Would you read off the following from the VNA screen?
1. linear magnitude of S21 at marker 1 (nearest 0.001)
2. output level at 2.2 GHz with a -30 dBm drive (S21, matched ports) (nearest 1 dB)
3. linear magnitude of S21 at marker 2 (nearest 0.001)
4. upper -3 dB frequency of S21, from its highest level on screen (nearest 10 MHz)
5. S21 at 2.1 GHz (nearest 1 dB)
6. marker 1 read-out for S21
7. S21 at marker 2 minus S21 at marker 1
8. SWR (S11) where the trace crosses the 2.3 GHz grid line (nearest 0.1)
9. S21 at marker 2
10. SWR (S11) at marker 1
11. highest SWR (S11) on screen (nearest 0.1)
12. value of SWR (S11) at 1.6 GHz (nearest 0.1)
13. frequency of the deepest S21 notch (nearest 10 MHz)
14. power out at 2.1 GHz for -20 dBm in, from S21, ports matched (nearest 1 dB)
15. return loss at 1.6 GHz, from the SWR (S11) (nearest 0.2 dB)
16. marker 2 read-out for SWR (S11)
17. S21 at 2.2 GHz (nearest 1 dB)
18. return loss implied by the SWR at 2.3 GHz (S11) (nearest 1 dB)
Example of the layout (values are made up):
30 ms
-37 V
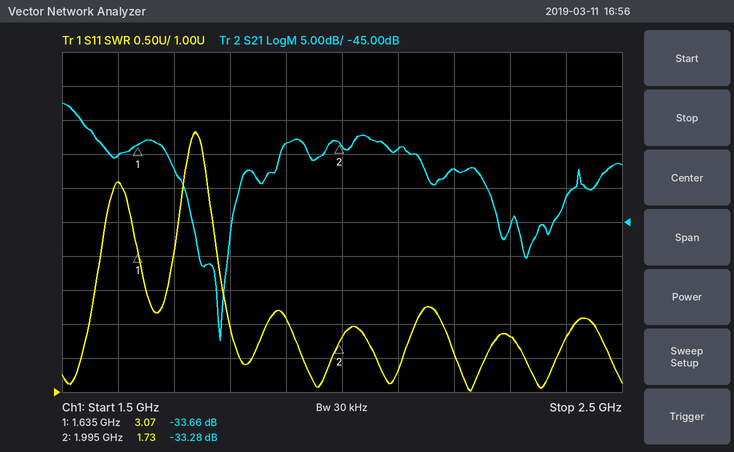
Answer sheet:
0.021
-67 dBm
0.022
1.54 GHz
-34 dB
-33.66 dB
0.38 dB
1.8
-33.28 dB
3.07
4.8
4.1
1.78 GHz
-54 dBm
4.4 dB
1.73
-37 dB
11 dB
